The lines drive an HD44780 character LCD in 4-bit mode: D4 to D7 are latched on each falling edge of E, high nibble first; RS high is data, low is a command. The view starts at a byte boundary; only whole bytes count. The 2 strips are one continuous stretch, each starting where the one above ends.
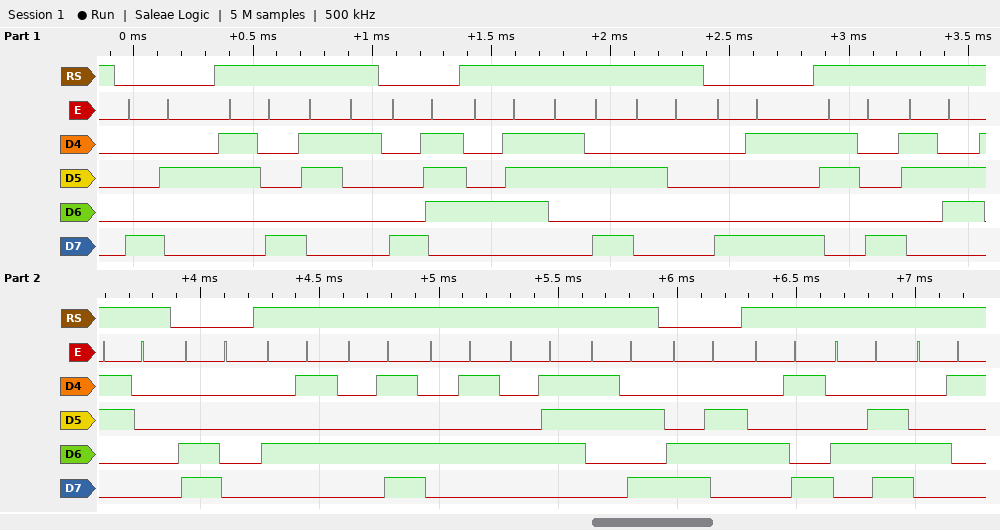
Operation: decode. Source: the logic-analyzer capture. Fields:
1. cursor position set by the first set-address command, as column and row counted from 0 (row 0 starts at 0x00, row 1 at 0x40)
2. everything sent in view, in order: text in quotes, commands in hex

column 2, row 0
0x82 "81" 0x87 "G: " 0x89 "860" 0xC0 "EMEG:" 0xC6 "INA"
